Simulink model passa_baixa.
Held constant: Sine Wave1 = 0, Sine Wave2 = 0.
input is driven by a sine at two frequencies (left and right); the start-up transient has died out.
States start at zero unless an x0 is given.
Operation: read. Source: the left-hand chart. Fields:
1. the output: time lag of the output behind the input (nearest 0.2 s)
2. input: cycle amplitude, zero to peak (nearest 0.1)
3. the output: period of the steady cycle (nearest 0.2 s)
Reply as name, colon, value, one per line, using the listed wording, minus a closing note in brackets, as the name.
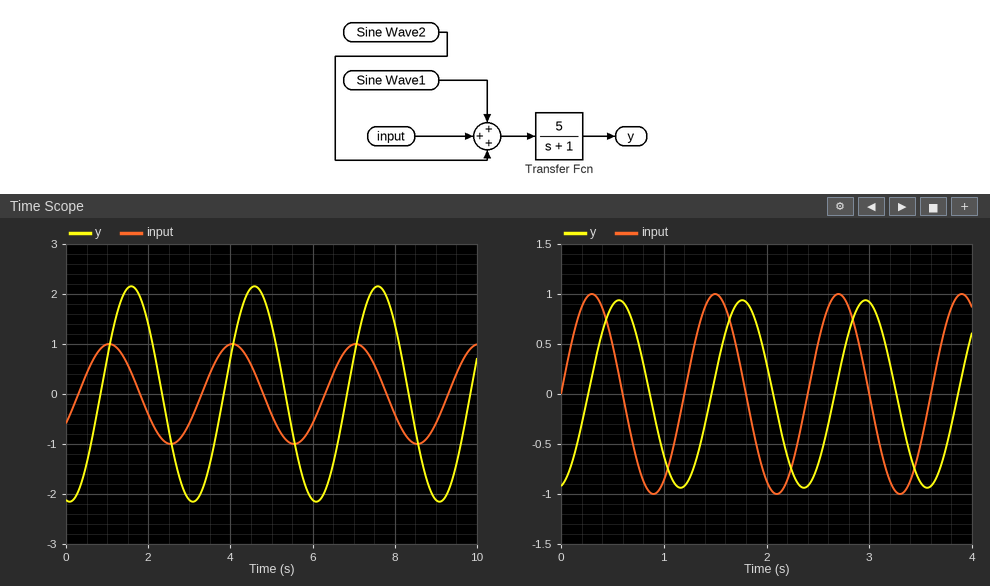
the output: time lag of the output behind the input: 0.6 s
input: cycle amplitude, zero to peak: 1.0
the output: period of the steady cycle: 3.0 s
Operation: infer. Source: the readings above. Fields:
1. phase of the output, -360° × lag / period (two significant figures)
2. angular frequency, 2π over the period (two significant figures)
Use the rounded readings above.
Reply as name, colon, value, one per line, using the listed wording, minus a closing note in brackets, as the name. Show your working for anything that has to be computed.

phase of the output, -360° × lag / period: -360 × 0.6 / 3 = -72°
angular frequency, 2π over the period: 2π / 3 = 2.1 rad/s
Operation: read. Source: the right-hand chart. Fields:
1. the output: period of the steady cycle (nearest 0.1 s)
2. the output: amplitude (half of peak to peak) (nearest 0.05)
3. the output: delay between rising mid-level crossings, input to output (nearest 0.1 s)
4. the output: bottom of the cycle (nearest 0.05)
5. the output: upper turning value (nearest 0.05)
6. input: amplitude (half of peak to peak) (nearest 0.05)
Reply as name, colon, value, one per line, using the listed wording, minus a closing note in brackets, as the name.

the output: period of the steady cycle: 1.2 s
the output: amplitude (half of peak to peak): 0.95
the output: delay between rising mid-level crossings, input to output: 0.3 s
the output: bottom of the cycle: -0.95
the output: upper turning value: 0.95
input: amplitude (half of peak to peak): 1.00
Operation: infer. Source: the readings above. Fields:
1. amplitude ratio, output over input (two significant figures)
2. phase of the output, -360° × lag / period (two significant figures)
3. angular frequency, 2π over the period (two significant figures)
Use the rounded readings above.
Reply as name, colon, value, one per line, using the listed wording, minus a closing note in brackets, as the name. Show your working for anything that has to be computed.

amplitude ratio, output over input: 0.95 / 1 = 0.95
phase of the output, -360° × lag / period: -360 × 0.3 / 1.2 = -90°
angular frequency, 2π over the period: 2π / 1.2 = 5.2 rad/s
